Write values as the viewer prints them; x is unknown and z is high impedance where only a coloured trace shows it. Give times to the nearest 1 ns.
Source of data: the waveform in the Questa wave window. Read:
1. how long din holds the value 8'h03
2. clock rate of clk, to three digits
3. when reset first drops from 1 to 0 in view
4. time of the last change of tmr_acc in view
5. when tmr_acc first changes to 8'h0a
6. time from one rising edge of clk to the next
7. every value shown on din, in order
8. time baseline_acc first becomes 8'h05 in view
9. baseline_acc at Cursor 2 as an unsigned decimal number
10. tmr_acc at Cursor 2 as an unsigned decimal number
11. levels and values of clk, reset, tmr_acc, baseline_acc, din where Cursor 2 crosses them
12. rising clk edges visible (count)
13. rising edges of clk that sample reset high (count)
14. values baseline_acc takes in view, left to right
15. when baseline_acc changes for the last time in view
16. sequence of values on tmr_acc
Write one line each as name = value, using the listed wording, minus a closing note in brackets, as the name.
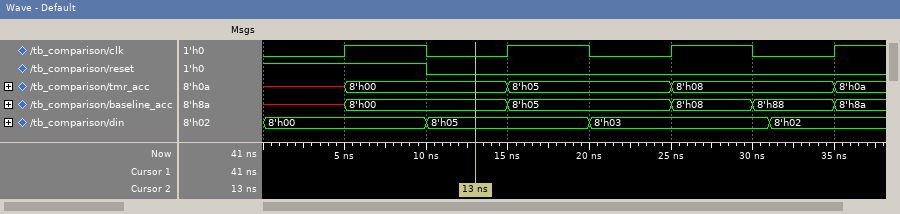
how long din holds the value 8'h03 = 11 ns
clock rate of clk, to three digits = 100 MHz
when reset first drops from 1 to 0 in view = 10 ns
time of the last change of tmr_acc in view = 35 ns
when tmr_acc first changes to 8'h0a = 35 ns
time from one rising edge of clk to the next = 10 ns
every value shown on din, in order = 8'h00, 8'h05, 8'h03, 8'h02
time baseline_acc first becomes 8'h05 in view = 15 ns
baseline_acc at Cursor 2 as an unsigned decimal number = 0
tmr_acc at Cursor 2 as an unsigned decimal number = 0
levels and values of clk, reset, tmr_acc, baseline_acc, din where Cursor 2 crosses them = clk=0, reset=0, tmr_acc=8'h00, baseline_acc=8'h00, din=8'h05
rising clk edges visible = 4
rising edges of clk that sample reset high = 1
values baseline_acc takes in view, left to right = x, 8'h00, 8'h05, 8'h08, 8'h88, 8'h8a
when baseline_acc changes for the last time in view = 35 ns
sequence of values on tmr_acc = x, 8'h00, 8'h05, 8'h08, 8'h0a
